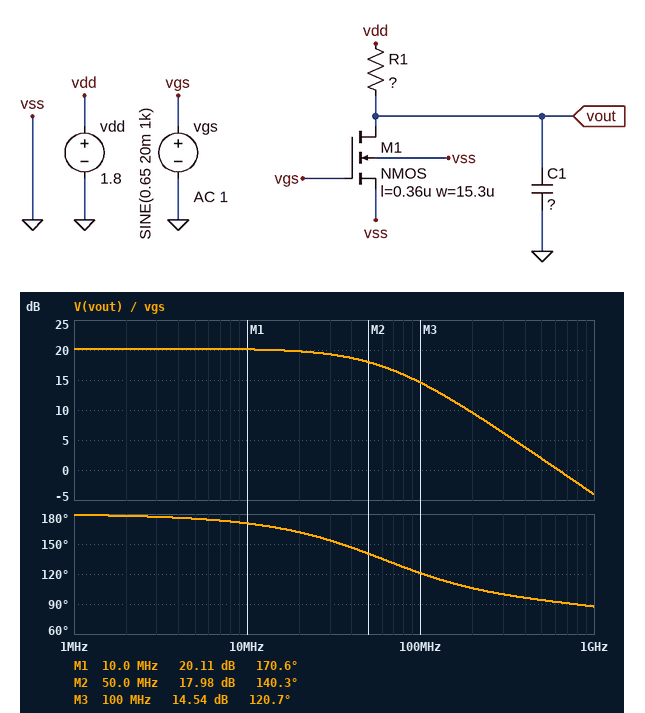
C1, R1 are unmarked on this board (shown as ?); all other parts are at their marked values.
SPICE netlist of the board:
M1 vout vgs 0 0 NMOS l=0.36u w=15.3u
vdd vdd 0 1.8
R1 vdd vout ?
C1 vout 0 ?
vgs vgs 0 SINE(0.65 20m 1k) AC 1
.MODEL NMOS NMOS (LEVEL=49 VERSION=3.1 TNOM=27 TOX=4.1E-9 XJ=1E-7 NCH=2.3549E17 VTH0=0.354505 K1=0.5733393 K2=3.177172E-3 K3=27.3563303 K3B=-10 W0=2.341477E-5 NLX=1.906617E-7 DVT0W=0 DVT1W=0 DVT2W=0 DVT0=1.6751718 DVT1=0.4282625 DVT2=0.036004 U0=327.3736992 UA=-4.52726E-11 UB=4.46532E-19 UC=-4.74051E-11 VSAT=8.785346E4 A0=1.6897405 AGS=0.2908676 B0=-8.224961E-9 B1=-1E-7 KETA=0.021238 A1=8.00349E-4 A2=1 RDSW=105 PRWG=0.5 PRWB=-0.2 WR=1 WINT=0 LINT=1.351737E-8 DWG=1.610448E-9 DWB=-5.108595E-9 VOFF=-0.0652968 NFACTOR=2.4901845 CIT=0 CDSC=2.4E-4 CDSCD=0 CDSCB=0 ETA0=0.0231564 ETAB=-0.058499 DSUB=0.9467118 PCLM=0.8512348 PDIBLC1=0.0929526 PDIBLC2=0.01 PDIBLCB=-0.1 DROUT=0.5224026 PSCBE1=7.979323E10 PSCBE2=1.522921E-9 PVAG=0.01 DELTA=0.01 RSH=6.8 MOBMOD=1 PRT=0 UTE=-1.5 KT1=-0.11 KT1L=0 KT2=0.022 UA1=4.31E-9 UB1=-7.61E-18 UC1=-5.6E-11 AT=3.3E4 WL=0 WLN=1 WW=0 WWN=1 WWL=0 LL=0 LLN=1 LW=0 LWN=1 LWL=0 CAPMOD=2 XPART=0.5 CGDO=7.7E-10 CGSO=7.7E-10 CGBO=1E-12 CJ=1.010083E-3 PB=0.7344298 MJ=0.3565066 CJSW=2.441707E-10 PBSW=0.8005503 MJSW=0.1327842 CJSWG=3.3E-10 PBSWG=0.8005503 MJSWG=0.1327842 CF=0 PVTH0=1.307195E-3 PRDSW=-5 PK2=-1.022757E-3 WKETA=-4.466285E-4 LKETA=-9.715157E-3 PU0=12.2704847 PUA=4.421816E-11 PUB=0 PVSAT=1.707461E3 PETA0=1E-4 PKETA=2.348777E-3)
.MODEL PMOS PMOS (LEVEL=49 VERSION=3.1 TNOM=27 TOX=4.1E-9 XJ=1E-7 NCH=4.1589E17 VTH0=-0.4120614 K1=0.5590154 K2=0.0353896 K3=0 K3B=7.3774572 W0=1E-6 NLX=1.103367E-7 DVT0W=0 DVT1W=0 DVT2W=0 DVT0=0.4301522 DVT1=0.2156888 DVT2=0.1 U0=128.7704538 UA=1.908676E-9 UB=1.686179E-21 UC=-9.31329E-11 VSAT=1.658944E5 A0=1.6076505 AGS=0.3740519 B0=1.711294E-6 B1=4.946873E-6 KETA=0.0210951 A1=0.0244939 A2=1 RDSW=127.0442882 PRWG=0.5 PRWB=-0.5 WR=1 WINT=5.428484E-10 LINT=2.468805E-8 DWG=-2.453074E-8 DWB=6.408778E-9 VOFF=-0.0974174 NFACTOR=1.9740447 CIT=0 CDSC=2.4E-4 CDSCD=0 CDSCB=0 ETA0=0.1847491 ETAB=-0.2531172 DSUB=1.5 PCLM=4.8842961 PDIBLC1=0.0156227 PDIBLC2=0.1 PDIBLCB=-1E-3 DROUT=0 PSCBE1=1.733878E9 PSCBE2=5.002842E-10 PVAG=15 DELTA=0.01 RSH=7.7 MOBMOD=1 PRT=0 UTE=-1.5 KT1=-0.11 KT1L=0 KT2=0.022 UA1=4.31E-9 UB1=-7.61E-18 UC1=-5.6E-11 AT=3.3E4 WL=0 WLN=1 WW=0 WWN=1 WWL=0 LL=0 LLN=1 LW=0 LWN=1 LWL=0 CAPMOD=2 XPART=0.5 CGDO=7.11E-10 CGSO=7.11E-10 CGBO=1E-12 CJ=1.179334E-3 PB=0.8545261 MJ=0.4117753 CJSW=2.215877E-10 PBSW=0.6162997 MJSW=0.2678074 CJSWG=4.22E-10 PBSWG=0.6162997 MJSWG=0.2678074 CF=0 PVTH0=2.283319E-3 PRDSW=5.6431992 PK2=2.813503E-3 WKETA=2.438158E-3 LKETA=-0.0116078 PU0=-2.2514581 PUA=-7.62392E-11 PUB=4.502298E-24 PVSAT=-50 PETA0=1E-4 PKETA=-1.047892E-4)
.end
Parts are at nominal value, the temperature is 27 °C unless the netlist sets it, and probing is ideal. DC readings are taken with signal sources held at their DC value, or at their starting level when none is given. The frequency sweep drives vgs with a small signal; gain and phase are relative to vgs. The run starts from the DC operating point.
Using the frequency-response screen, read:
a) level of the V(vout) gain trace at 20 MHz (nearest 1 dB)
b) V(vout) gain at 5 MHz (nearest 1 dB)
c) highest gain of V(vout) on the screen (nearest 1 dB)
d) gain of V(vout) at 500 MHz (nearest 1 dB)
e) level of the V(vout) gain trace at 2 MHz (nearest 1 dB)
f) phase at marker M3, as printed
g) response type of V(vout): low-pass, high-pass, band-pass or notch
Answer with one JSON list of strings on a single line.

["20 dB", "20 dB", "20 dB", "2 dB", "20 dB", "120.7 deg", "low-pass"]
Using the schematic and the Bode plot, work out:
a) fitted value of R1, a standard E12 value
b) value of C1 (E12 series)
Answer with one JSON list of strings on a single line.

["12 kΩ", "390 fF"]
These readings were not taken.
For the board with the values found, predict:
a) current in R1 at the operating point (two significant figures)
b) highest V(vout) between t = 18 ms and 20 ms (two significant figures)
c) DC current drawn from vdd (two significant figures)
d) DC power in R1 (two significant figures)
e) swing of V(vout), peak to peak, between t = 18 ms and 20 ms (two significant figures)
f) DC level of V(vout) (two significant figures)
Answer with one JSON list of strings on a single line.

["130 µA", "480 mV", "130 µA", "210 µW", "370 mV", "200 mV"]
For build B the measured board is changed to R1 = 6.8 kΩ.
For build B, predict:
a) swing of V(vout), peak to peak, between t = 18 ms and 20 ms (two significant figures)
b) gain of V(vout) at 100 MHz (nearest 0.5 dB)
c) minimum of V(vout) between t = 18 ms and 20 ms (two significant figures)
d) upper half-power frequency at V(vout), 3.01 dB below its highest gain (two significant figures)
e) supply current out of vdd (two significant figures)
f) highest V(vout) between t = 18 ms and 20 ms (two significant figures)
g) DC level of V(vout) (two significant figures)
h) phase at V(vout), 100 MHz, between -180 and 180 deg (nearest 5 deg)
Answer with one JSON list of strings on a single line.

["430 mV", "15.5 dB", "570 mV", "64 MHz", "150 µA", "1.0 V", "800 mV", "120 deg"]
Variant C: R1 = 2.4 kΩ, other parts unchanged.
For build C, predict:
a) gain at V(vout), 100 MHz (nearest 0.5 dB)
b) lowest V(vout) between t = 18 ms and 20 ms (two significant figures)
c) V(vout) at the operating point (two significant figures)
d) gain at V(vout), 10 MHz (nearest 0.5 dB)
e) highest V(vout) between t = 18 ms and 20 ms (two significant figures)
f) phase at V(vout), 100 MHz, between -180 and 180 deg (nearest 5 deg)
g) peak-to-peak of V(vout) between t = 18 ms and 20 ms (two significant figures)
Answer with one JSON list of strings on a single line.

["11.5 dB", "1.3 V", "1.4 V", "12.5 dB", "1.5 V", "150 deg", "170 mV"]
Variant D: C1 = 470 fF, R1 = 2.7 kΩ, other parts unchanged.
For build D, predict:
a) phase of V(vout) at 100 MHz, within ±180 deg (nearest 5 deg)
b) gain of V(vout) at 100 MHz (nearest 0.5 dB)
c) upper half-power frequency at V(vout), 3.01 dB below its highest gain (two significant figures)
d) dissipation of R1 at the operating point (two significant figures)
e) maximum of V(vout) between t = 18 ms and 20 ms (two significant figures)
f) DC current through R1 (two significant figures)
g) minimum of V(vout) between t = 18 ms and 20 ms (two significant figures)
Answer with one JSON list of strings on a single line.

["140 deg", "11.5 dB", "130 MHz", "66 µW", "1.5 V", "160 µA", "1.3 V"]
